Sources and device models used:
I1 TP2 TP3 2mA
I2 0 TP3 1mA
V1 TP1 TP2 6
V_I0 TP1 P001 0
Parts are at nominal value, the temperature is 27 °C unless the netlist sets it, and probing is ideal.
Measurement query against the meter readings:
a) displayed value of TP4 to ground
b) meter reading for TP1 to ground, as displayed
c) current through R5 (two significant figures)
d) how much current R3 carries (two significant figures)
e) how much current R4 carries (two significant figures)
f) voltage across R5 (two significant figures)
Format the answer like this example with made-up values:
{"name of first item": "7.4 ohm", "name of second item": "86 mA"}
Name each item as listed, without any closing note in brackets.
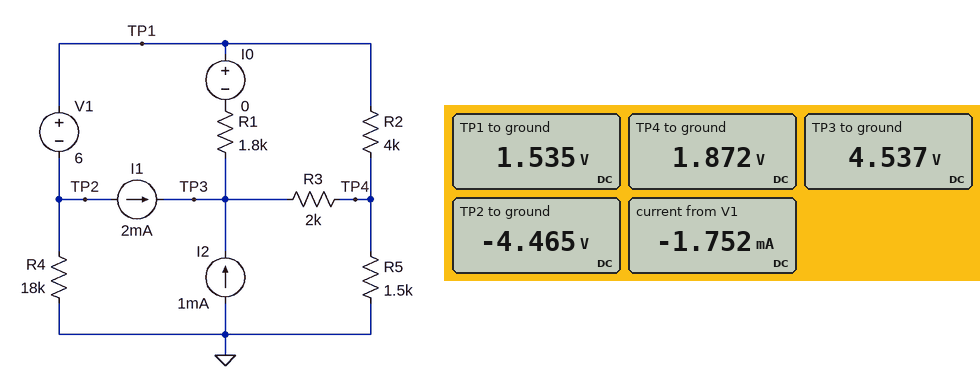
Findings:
{"displayed value of TP4 to ground": "1.872 V", "meter reading for TP1 to ground, as displayed": "1.535 V", "current through R5": "1.2 mA", "how much current R3 carries": "1.3 mA", "how much current R4 carries": "250 µA", "voltage across R5": "1.9 V"}
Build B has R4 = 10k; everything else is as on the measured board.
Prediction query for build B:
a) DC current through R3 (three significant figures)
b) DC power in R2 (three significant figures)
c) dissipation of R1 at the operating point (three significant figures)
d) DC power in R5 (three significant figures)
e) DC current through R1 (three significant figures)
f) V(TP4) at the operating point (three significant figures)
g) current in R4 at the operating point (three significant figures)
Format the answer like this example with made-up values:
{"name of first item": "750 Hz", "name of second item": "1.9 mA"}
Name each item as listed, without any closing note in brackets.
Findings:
{"DC current through R3": "1.41 mA", "DC power in R2": "614 nW", "dissipation of R1 at the operating point": "4.56 mW", "DC power in R5": "2.92 mW", "DC current through R1": "1.59 mA", "V(TP4) at the operating point": "2.09 V", "current in R4 at the operating point": "396 µA"}
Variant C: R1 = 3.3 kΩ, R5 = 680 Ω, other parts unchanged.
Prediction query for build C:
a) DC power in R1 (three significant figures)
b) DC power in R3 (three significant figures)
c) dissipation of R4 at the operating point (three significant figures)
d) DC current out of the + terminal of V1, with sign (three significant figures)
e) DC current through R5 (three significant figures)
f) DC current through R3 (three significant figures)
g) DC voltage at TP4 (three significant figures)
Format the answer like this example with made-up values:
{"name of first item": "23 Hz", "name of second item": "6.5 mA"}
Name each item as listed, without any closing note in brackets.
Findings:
{"DC power in R1": "6.06 mW", "DC power in R3": "5.41 mW", "dissipation of R4 at the operating point": "2.18 mW", "DC current out of the + terminal of V1, with sign": "-1.65 mA", "DC current through R5": "1.35 mA", "DC current through R3": "1.64 mA", "DC voltage at TP4": "917 mV"}
